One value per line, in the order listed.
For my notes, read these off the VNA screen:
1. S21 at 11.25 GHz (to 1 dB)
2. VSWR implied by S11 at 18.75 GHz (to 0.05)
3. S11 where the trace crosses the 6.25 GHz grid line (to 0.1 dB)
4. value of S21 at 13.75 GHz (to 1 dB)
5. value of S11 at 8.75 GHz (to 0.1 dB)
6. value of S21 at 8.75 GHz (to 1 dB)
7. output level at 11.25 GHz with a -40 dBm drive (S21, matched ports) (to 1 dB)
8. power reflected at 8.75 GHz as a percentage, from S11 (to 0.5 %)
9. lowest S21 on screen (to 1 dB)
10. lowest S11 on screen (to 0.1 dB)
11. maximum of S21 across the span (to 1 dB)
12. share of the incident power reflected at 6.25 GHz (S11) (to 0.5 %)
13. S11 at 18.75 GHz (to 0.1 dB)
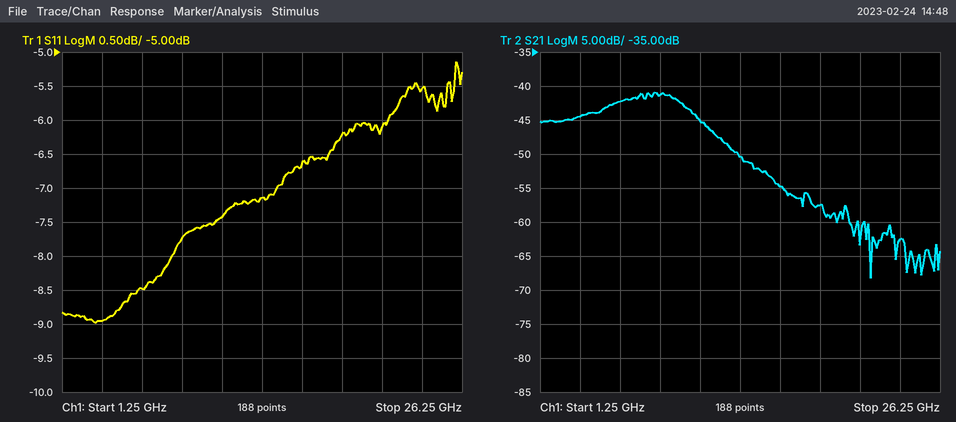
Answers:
-45 dB
2.90
-8.5 dB
-50 dB
-7.7 dB
-41 dB
-85 dBm
17.0 %
-68 dB
-9.0 dB
-41 dB
14.0 %
-6.2 dB
